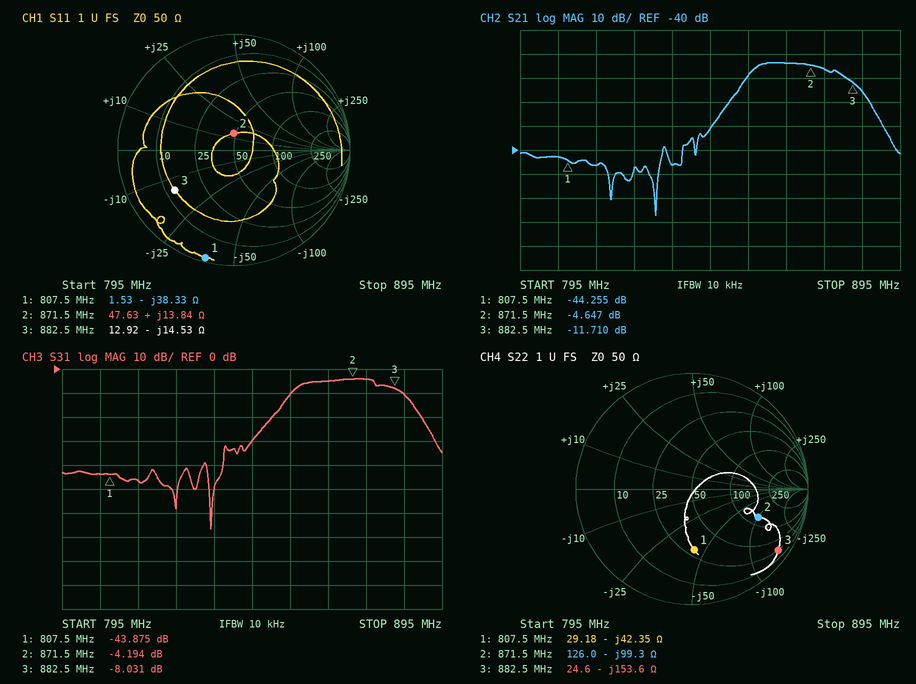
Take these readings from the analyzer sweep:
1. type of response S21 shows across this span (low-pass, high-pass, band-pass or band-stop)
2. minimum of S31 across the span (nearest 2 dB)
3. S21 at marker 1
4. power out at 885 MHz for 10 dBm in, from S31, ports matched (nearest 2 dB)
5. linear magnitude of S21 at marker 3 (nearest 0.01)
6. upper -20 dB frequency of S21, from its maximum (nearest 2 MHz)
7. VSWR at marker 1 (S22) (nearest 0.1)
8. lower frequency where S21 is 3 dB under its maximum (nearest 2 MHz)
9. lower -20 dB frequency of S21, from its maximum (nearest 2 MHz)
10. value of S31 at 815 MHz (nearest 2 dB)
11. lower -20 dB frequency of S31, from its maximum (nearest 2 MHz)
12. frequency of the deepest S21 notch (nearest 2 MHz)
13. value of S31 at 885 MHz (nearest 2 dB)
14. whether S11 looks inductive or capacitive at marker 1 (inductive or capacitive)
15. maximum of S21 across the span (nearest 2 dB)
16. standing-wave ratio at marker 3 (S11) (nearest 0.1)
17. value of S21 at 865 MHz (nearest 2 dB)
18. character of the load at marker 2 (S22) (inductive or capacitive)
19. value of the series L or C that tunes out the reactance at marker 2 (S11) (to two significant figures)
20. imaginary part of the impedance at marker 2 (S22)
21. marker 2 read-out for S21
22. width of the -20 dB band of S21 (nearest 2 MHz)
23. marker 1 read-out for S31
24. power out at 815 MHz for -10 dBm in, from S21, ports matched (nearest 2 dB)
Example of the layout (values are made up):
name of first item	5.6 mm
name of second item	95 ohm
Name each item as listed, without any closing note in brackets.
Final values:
type of response S21 shows across this span	band-pass
minimum of S31 across the span	-66 dB
S21 at marker 1	-44.255 dB
power out at 885 MHz for 10 dBm in, from S31, ports matched	0 dBm
linear magnitude of S21 at marker 3	0.26
upper -20 dB frequency of S21, from its maximum	888 MHz
VSWR at marker 1 (S22)	3.2
lower frequency where S21 is 3 dB under its maximum	856 MHz
lower -20 dB frequency of S21, from its maximum	848 MHz
value of S31 at 815 MHz	-46 dB
lower -20 dB frequency of S31, from its maximum	848 MHz
frequency of the deepest S21 notch	830 MHz
value of S31 at 885 MHz	-10 dB
whether S11 looks inductive or capacitive at marker 1	capacitive
maximum of S21 across the span	-4 dB
standing-wave ratio at marker 3 (S11)	4.2
value of S21 at 865 MHz	-4 dB
character of the load at marker 2 (S22)	capacitive
value of the series L or C that tunes out the reactance at marker 2 (S11)	13 pF
imaginary part of the impedance at marker 2	-99.3 Ω
marker 2 read-out for S21	-4.647 dB
width of the -20 dB band of S21	40 MHz
marker 1 read-out for S31	-43.875 dB
power out at 815 MHz for -10 dBm in, from S21, ports matched	-56 dBm
